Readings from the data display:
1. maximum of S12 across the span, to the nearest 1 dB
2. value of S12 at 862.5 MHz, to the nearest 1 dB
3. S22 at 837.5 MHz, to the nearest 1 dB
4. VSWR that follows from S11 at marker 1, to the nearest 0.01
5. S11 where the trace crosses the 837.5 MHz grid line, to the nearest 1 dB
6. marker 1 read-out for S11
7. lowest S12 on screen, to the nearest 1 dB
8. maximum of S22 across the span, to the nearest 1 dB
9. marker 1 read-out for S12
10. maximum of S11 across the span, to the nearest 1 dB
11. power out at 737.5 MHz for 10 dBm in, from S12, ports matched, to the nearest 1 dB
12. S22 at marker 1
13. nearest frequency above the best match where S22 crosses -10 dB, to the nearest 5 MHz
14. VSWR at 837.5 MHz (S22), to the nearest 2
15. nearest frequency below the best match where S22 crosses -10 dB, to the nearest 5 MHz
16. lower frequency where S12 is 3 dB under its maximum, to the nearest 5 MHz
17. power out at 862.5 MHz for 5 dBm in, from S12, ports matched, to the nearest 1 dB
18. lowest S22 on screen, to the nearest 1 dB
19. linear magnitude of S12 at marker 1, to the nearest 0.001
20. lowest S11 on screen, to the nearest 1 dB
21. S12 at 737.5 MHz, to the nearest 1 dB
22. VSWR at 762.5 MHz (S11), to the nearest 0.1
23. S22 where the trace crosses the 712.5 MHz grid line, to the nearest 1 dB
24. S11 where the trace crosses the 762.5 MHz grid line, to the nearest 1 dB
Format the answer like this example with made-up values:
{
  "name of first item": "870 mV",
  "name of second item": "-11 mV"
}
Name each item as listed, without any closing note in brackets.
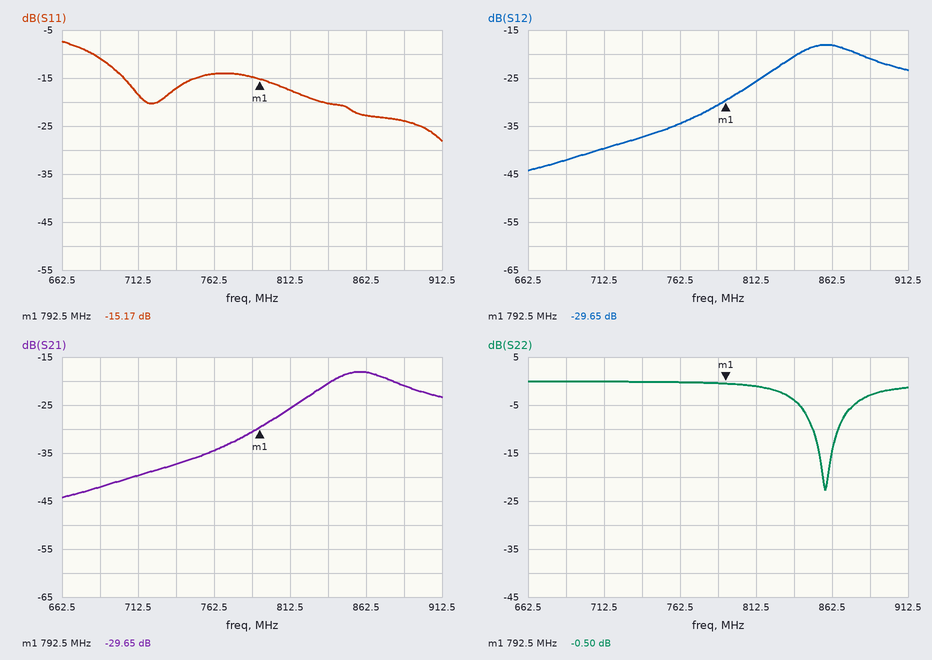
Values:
{
  "maximum of S12 across the span, to the nearest 1 dB": "-18 dB",
  "value of S12 at 862.5 MHz, to the nearest 1 dB": "-18 dB",
  "S22 at 837.5 MHz, to the nearest 1 dB": "-4 dB",
  "VSWR that follows from S11 at marker 1, to the nearest 0.01": "1.42",
  "S11 where the trace crosses the 837.5 MHz grid line, to the nearest 1 dB": "-20 dB",
  "marker 1 read-out for S11": "-15.17 dB",
  "lowest S12 on screen, to the nearest 1 dB": "-44 dB",
  "maximum of S22 across the span, to the nearest 1 dB": "0 dB",
  "marker 1 read-out for S12": "-29.65 dB",
  "maximum of S11 across the span, to the nearest 1 dB": "-7 dB",
  "power out at 737.5 MHz for 10 dBm in, from S12, ports matched, to the nearest 1 dB": "-27 dBm",
  "S22 at marker 1": "-0.50 dB",
  "nearest frequency above the best match where S22 crosses -10 dB, to the nearest 5 MHz": "865 MHz",
  "VSWR at 837.5 MHz (S22), to the nearest 2": "4",
  "nearest frequency below the best match where S22 crosses -10 dB, to the nearest 5 MHz": "850 MHz",
  "lower frequency where S12 is 3 dB under its maximum, to the nearest 5 MHz": "835 MHz",
  "power out at 862.5 MHz for 5 dBm in, from S12, ports matched, to the nearest 1 dB": "-13 dBm",
  "lowest S22 on screen, to the nearest 1 dB": "-23 dB",
  "linear magnitude of S12 at marker 1, to the nearest 0.001": "0.033",
  "lowest S11 on screen, to the nearest 1 dB": "-28 dB",
  "S12 at 737.5 MHz, to the nearest 1 dB": "-37 dB",
  "VSWR at 762.5 MHz (S11), to the nearest 0.1": "1.5",
  "S22 where the trace crosses the 712.5 MHz grid line, to the nearest 1 dB": "0 dB",
  "S11 where the trace crosses the 762.5 MHz grid line, to the nearest 1 dB": "-14 dB"
}
